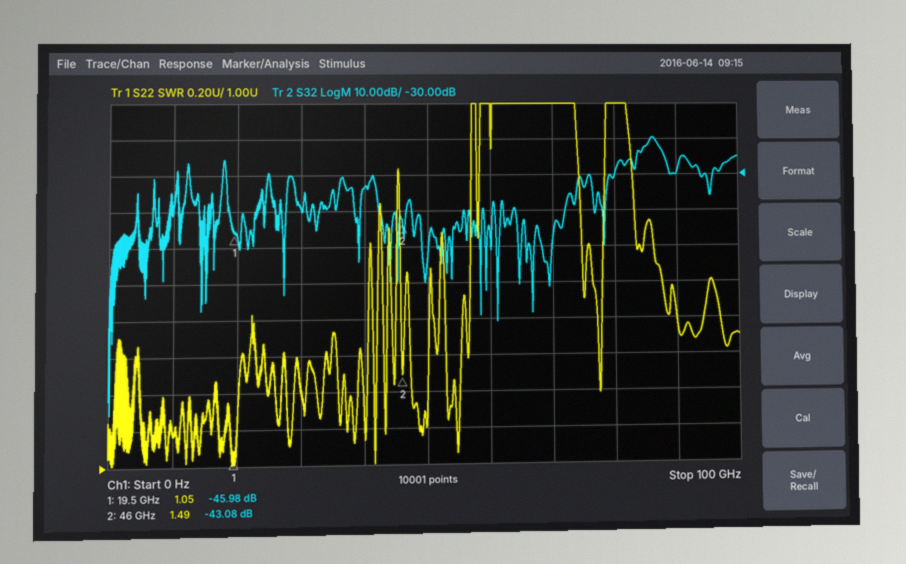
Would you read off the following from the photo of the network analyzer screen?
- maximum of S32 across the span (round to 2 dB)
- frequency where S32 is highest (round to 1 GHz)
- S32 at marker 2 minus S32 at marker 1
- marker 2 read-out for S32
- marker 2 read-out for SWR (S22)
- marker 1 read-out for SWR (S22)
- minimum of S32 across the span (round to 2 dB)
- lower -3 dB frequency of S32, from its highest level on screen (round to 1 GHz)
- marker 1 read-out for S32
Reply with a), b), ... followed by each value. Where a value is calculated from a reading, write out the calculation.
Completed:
a) -20 dB
b) 86 GHz
c) -43.08 − (-45.98) = 2.90 dB
d) -43.08 dB
e) 1.49
f) 1.05
g) -96 dB
h) 85 GHz
i) -45.98 dB
